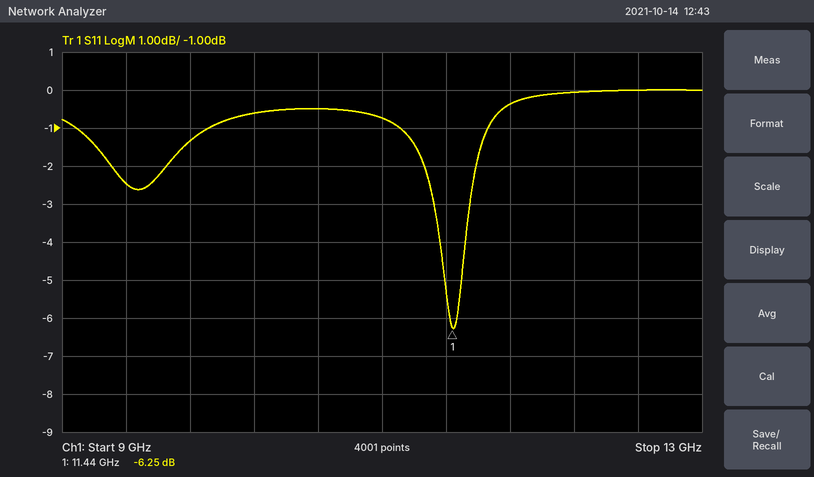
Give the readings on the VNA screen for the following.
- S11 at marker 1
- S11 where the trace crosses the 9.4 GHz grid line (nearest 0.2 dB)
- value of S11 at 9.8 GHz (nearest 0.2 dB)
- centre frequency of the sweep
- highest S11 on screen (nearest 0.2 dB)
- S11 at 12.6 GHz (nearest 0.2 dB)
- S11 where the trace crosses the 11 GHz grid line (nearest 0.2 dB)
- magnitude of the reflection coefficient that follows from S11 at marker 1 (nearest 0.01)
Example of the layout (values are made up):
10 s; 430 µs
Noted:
-6.25 dB; -2.4 dB; -1.4 dB; 11 GHz; 0.0 dB; 0.0 dB; -0.8 dB; 0.49
